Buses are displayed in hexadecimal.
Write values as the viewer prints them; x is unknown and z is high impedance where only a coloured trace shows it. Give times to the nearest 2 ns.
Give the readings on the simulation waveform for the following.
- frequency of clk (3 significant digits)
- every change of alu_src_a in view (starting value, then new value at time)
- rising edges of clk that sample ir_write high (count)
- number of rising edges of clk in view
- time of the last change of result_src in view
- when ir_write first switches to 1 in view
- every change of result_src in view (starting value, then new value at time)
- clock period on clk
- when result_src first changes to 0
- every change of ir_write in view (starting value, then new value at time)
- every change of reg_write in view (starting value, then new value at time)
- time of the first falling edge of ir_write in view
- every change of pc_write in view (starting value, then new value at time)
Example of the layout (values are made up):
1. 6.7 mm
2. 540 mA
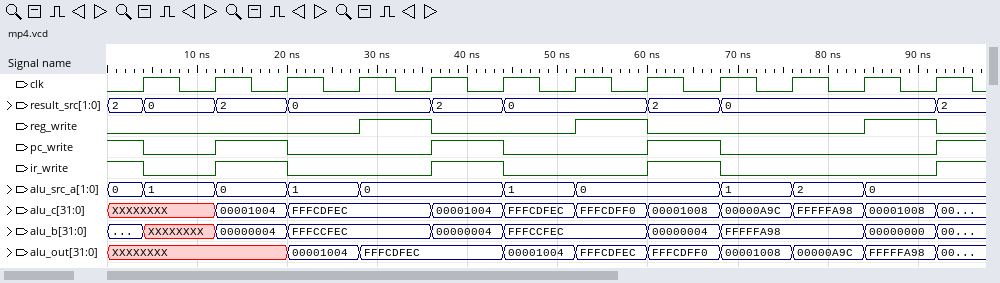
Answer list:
1. 125 MHz
2. 0, 1 at 4 ns, 0 at 12 ns, 1 at 20 ns, 0 at 28 ns, 1 at 44 ns, 0 at 52 ns, 1 at 68 ns, 2 at 76 ns, 0 at 84 ns
3. 4
4. 12
5. 92 ns
6. 12 ns
7. 2, 0 at 4 ns, 2 at 12 ns, 0 at 20 ns, 2 at 36 ns, 0 at 44 ns, 2 at 60 ns, 0 at 68 ns, 2 at 92 ns
8. 8 ns
9. 4 ns
10. 1, 0 at 4 ns, 1 at 12 ns, 0 at 20 ns, 1 at 36 ns, 0 at 44 ns, 1 at 60 ns, 0 at 68 ns, 1 at 92 ns
11. 0, 1 at 28 ns, 0 at 36 ns, 1 at 52 ns, 0 at 60 ns, 1 at 84 ns, 0 at 92 ns
12. 4 ns
13. 1, 0 at 4 ns, 1 at 12 ns, 0 at 20 ns, 1 at 36 ns, 0 at 44 ns, 1 at 60 ns, 0 at 68 ns, 1 at 92 ns
